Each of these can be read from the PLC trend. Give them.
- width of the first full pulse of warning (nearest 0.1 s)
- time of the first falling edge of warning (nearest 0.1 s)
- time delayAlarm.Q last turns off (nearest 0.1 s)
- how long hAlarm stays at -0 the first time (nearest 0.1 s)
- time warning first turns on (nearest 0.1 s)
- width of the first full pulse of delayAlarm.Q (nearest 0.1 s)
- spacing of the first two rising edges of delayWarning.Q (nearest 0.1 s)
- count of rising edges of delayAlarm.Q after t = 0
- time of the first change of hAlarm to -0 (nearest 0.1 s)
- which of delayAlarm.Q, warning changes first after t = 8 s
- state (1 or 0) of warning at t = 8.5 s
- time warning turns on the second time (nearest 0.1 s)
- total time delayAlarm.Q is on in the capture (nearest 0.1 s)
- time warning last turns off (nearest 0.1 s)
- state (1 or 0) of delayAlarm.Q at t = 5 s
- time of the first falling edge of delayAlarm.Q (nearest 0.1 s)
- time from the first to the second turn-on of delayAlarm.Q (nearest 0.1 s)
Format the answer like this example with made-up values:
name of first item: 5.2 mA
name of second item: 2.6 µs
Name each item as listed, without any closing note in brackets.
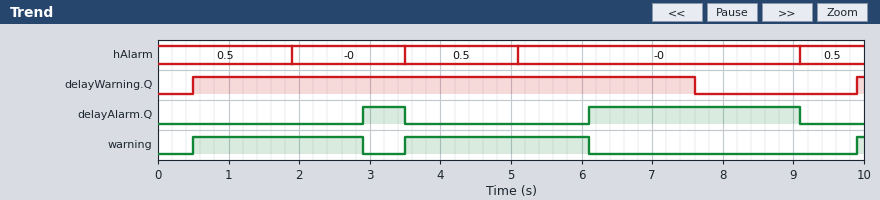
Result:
width of the first full pulse of warning: 2.4 s
time of the first falling edge of warning: 2.9 s
time delayAlarm.Q last turns off: 9.1 s
how long hAlarm stays at -0 the first time: 1.6 s
time warning first turns on: 0.5 s
width of the first full pulse of delayAlarm.Q: 0.6 s
spacing of the first two rising edges of delayWarning.Q: 9.4 s
count of rising edges of delayAlarm.Q after t = 0: 2
time of the first change of hAlarm to -0: 1.9 s
which of delayAlarm.Q, warning changes first after t = 8 s: delayAlarm.Q
state (1 or 0) of warning at t = 8.5 s: 0
time warning turns on the second time: 3.5 s
total time delayAlarm.Q is on in the capture: 3.6 s
time warning last turns off: 6.1 s
state (1 or 0) of delayAlarm.Q at t = 5 s: 0
time of the first falling edge of delayAlarm.Q: 3.5 s
time from the first to the second turn-on of delayAlarm.Q: 3.2 s
